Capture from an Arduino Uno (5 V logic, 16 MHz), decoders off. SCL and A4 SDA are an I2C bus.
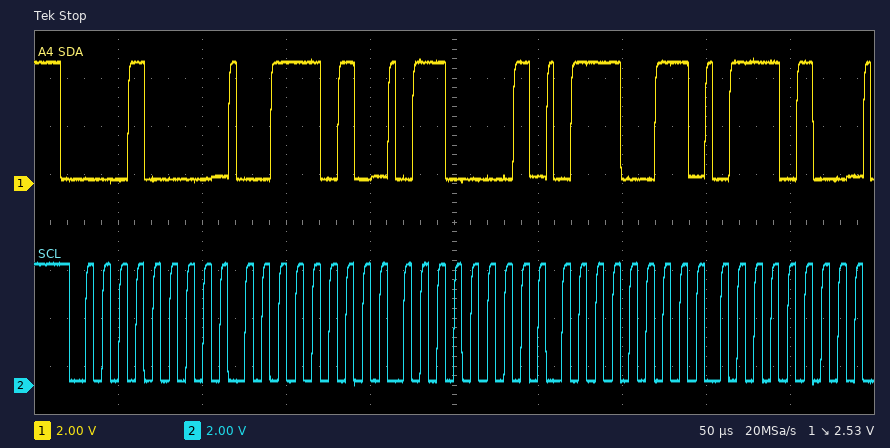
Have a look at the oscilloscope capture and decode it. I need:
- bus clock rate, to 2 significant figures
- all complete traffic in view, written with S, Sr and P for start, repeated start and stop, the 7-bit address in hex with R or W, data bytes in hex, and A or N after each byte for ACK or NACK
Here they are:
100 kHz
S 08W A 3A A 61 A 73 A 74 A
